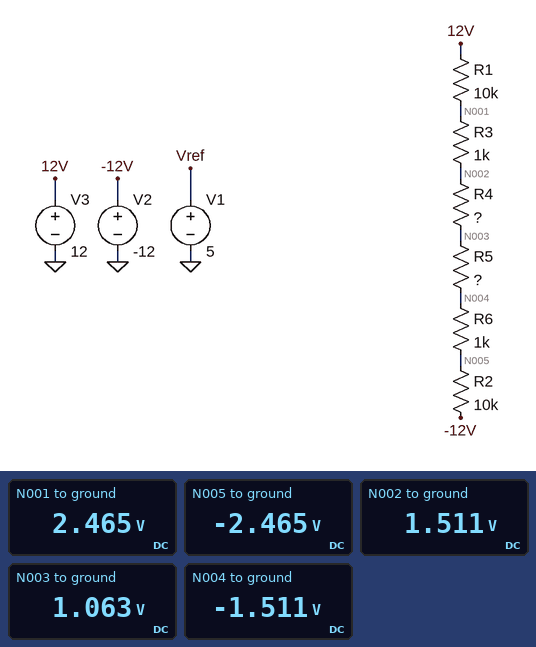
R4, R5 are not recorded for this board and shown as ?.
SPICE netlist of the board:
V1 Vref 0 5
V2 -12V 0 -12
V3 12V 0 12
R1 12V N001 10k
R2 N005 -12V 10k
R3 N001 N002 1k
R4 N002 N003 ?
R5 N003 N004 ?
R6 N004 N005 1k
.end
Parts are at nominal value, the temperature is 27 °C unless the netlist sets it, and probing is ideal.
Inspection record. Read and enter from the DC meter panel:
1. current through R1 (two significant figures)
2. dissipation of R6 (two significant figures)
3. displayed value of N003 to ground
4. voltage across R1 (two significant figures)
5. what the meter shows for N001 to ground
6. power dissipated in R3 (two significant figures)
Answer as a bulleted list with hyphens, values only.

- 950 µA
- 910 µW
- 1.063 V
- 9.5 V
- 2.465 V
- 910 µW
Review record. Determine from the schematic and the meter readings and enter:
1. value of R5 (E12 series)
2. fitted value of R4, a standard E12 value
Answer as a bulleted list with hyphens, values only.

- 2.7 kΩ
- 470 Ω
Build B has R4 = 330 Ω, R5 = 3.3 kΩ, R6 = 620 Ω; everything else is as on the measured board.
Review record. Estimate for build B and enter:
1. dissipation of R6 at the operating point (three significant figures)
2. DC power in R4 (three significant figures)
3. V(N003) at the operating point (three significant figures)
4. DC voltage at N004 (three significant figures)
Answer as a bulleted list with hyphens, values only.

- 560 µW
- 298 µW
- 1.23 V
- -1.91 V
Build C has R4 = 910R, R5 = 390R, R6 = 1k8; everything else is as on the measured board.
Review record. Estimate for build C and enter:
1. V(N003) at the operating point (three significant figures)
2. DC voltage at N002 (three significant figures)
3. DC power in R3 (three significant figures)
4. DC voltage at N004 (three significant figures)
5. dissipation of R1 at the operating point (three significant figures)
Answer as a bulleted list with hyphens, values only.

- 139 mV
- 1.05 V
- 992 µW
- -249 mV
- 9.92 mW
